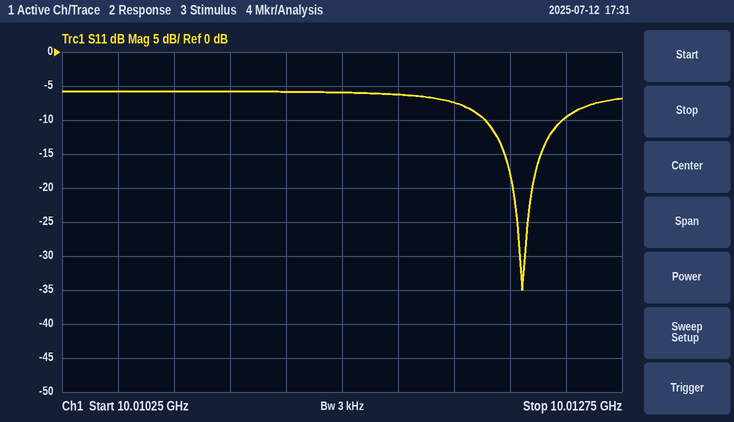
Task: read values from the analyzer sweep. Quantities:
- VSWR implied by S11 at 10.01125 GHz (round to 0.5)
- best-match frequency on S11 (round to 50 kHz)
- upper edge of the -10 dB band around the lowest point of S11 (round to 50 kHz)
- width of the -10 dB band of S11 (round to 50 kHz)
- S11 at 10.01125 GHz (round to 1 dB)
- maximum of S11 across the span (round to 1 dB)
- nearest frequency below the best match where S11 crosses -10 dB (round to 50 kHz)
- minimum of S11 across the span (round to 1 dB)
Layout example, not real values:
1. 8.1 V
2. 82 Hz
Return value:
1. 3.0
2. 10.01230 GHz
3. 10.01250 GHz
4. 350 kHz
5. -6 dB
6. -6 dB
7. 10.01215 GHz
8. -35 dB
